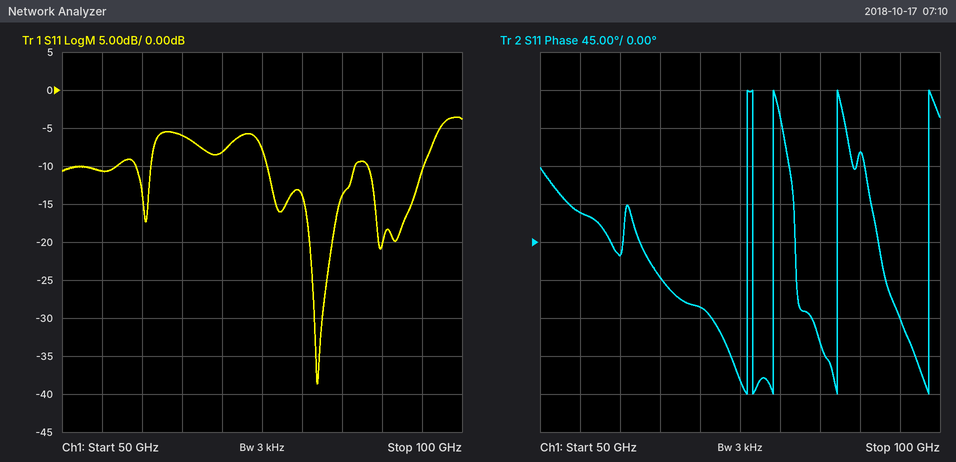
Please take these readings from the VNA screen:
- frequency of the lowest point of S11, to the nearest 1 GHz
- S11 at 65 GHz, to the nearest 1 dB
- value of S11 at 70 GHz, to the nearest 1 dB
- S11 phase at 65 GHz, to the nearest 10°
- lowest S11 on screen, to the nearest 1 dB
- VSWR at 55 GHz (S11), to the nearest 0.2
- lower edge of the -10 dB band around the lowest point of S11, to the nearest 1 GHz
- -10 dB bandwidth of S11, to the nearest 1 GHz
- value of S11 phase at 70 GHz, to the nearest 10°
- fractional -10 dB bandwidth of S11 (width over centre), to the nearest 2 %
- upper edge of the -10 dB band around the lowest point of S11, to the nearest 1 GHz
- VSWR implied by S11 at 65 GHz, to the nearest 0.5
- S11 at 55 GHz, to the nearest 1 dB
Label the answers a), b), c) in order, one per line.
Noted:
a) 82 GHz
b) -6 dB
c) -8 dB
d) -40°
e) -39 dB
f) 1.8
g) 76 GHz
h) 11 GHz
i) -80°
j) 14 %
k) 87 GHz
l) 3.0
m) -11 dB
